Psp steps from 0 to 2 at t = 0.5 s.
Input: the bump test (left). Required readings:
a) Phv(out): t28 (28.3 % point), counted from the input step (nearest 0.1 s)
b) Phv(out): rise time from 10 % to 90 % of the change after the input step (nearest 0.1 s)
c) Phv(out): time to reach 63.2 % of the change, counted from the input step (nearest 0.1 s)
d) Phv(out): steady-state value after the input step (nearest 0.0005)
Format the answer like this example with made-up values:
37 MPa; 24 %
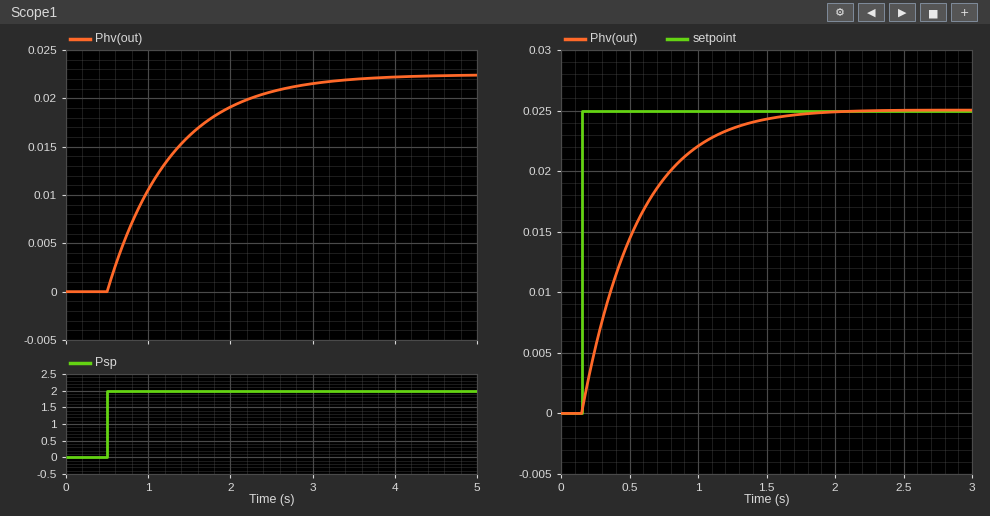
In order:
0.3 s; 1.7 s; 0.8 s; 0.0225
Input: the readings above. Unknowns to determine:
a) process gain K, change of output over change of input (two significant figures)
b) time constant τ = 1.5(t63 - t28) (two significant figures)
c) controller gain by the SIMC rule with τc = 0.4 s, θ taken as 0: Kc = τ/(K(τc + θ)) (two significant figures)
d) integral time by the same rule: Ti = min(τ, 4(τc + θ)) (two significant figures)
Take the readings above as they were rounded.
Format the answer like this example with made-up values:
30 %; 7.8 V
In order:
0.011; 0.75 s; 170; 0.75 s
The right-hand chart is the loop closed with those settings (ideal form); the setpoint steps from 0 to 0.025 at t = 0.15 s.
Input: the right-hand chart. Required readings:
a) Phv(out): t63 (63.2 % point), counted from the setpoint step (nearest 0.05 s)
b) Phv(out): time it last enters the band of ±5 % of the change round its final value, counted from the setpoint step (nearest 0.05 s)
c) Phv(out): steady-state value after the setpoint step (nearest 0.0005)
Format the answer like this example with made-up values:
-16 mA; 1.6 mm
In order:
0.40 s; 1.15 s; 0.0250
